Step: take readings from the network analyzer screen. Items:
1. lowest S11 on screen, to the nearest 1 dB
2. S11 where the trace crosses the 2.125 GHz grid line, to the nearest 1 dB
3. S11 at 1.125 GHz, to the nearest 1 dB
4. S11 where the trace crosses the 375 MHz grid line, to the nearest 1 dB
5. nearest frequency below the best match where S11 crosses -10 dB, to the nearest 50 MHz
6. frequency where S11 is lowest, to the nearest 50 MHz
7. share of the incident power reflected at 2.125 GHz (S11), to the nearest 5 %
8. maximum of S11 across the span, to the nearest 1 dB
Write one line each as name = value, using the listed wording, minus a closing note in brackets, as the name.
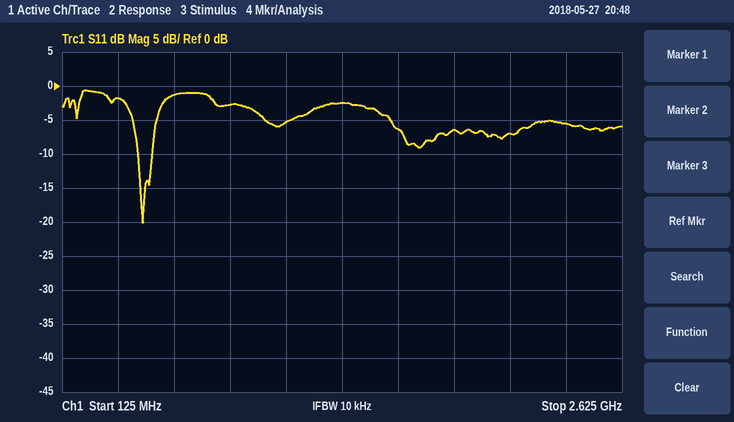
lowest S11 on screen, to the nearest 1 dB = -20 dB
S11 where the trace crosses the 2.125 GHz grid line, to the nearest 1 dB = -7 dB
S11 at 1.125 GHz, to the nearest 1 dB = -5 dB
S11 where the trace crosses the 375 MHz grid line, to the nearest 1 dB = -2 dB
nearest frequency below the best match where S11 crosses -10 dB, to the nearest 50 MHz = 450 MHz
frequency where S11 is lowest, to the nearest 50 MHz = 500 MHz
share of the incident power reflected at 2.125 GHz (S11), to the nearest 5 % = 20 %
maximum of S11 across the span, to the nearest 1 dB = -1 dB
